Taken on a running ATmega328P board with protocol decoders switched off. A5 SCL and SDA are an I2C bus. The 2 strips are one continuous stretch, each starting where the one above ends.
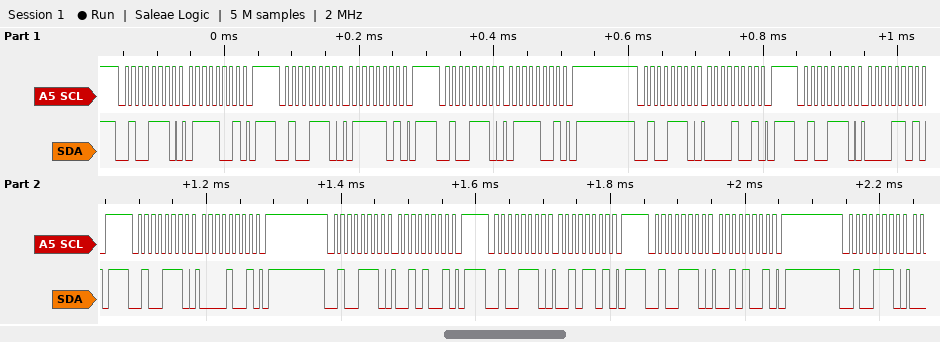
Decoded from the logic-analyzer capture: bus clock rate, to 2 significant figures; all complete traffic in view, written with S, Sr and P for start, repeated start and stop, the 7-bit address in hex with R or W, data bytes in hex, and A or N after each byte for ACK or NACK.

100 kHz
S 27W A 79 A P S 27W A 7D A P S 27W A 79 A P S 27W A 09 A P S 27W A 0D A P S 27W A 09 A P S 27W A 29 A P S 27W A 2D A P S 27W A 29 A P S 27W A
